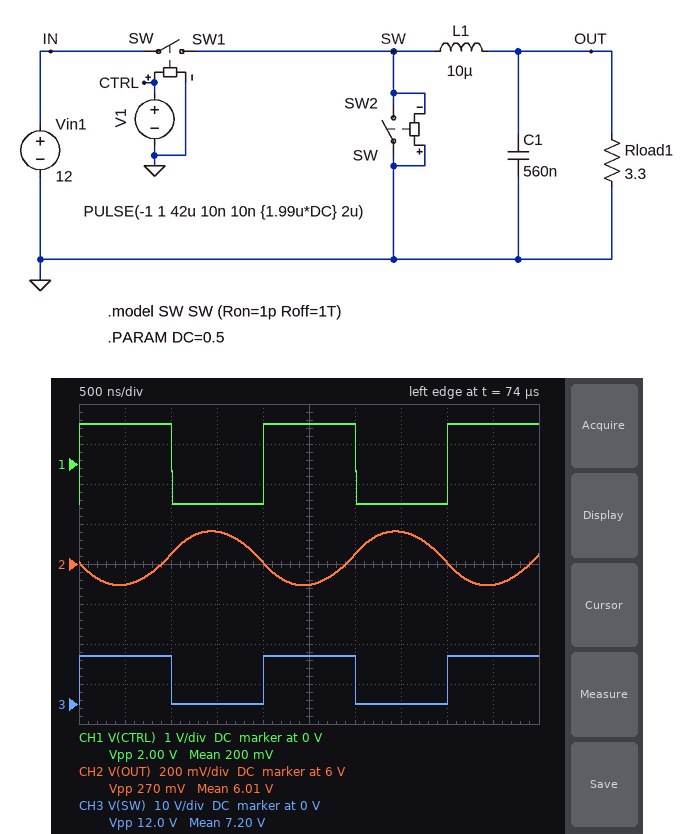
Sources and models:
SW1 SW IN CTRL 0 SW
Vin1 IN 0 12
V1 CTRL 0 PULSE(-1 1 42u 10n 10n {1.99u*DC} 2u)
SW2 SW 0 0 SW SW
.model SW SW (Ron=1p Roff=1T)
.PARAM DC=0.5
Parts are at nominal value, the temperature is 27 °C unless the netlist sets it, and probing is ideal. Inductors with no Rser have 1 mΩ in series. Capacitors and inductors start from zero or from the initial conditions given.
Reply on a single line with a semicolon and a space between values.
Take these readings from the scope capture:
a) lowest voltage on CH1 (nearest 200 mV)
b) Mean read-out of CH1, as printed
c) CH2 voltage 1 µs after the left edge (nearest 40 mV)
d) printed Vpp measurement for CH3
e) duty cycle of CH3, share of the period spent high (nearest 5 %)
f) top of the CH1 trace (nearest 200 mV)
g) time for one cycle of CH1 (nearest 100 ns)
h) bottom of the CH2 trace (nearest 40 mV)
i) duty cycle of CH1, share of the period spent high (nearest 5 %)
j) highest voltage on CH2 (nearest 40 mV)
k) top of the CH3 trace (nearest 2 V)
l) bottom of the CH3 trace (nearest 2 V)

-1.0 V; 200 mV; 6.04 V; 12.0 V; 50 %; 1.0 V; 2.0 µs; 5.88 V; 50 %; 6.16 V; 12 V; 0 V
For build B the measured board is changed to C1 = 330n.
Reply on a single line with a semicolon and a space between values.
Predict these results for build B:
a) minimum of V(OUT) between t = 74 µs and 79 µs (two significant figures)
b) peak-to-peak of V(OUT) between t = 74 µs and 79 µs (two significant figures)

5.8 V; 450 mV
